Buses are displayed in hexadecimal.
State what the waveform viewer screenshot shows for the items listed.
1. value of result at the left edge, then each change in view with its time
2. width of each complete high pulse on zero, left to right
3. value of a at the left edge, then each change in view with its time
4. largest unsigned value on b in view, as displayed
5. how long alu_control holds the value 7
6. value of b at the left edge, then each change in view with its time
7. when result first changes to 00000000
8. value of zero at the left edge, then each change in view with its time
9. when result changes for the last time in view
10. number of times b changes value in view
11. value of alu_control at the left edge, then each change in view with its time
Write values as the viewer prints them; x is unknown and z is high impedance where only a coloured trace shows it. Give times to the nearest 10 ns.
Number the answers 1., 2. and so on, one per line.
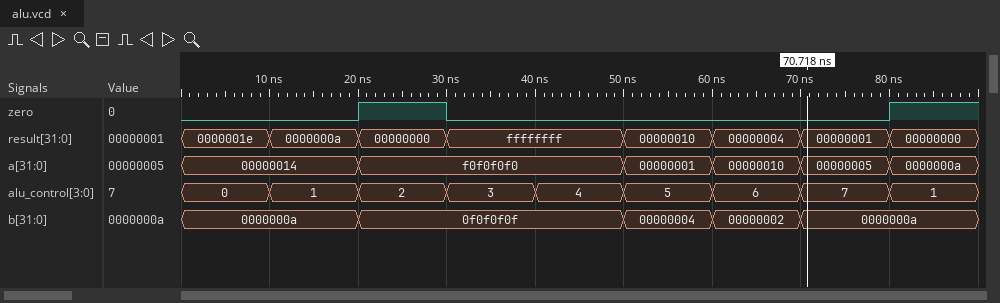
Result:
1. 0000001e, 0000000a at 10 ns, 00000000 at 20 ns, ffffffff at 30 ns, 00000010 at 50 ns, 00000004 at 60 ns, 00000001 at 70 ns, 00000000 at 80 ns
2. 10 ns
3. 00000014, f0f0f0f0 at 20 ns, 00000001 at 50 ns, 00000010 at 60 ns, 00000005 at 70 ns, 0000000a at 80 ns
4. 0f0f0f0f
5. 10 ns
6. 0000000a, 0f0f0f0f at 20 ns, 00000004 at 50 ns, 00000002 at 60 ns, 0000000a at 70 ns
7. 20 ns
8. 0, 1 at 20 ns, 0 at 30 ns, 1 at 80 ns
9. 80 ns
10. 4
11. 0, 1 at 10 ns, 2 at 20 ns, 3 at 30 ns, 4 at 40 ns, 5 at 50 ns, 6 at 60 ns, 7 at 70 ns, 1 at 80 ns
